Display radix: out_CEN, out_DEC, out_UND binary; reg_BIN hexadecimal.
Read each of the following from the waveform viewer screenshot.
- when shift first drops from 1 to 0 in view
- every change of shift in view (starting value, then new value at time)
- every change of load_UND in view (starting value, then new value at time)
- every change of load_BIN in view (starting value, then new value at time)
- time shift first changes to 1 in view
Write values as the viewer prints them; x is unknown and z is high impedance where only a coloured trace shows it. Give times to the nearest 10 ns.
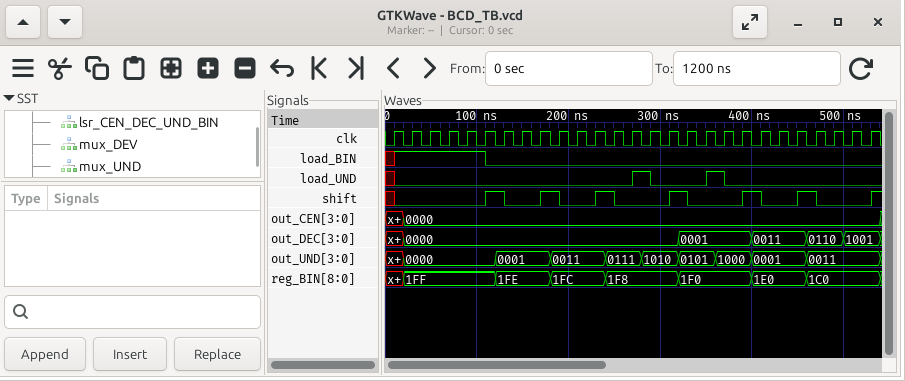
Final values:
130 ns
x, 0 at 10 ns, 1 at 110 ns, 0 at 130 ns, 1 at 170 ns, 0 at 190 ns, 1 at 230 ns, 0 at 250 ns, 1 at 310 ns, 0 at 330 ns, 1 at 390 ns, 0 at 410 ns, 1 at 450 ns, 0 at 470 ns, 1 at 530 ns
x, 0 at 10 ns, 1 at 270 ns, 0 at 290 ns, 1 at 350 ns, 0 at 370 ns
x, 1 at 10 ns, 0 at 110 ns
110 ns
